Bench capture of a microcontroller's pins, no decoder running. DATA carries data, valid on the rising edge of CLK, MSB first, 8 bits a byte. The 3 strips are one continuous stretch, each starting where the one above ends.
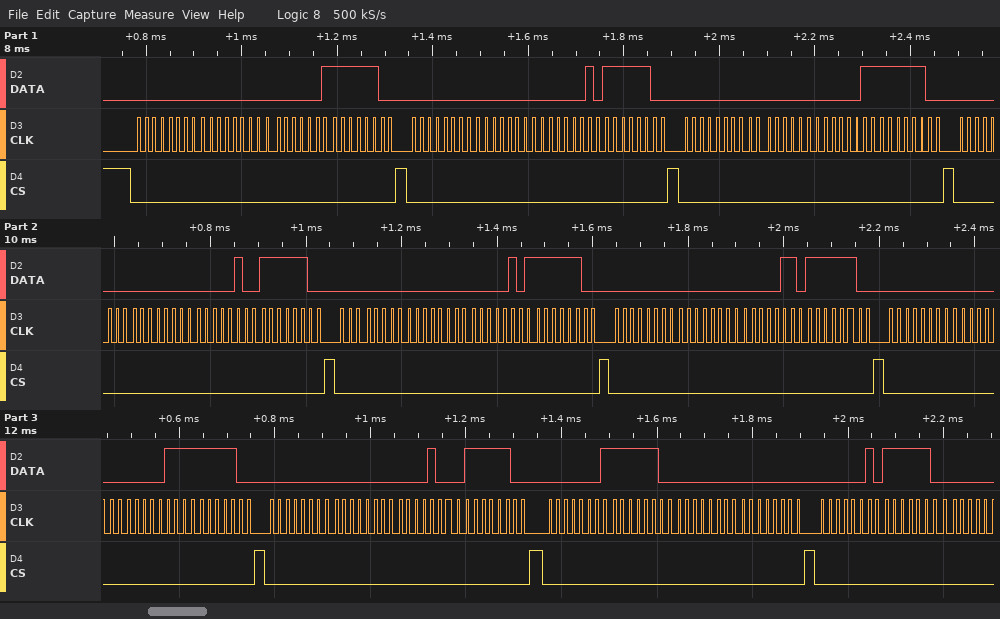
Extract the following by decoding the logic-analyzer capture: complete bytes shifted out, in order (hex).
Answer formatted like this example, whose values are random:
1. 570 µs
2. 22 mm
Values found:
1. 00 00 01 FC 00 00 02 FC 00 00 03 FC 00 00 04 FC 00 00 05 FC 00 00 06 FC 00 00 07 FC 00 00 08 FC 01 FC 00 00 02 FC
